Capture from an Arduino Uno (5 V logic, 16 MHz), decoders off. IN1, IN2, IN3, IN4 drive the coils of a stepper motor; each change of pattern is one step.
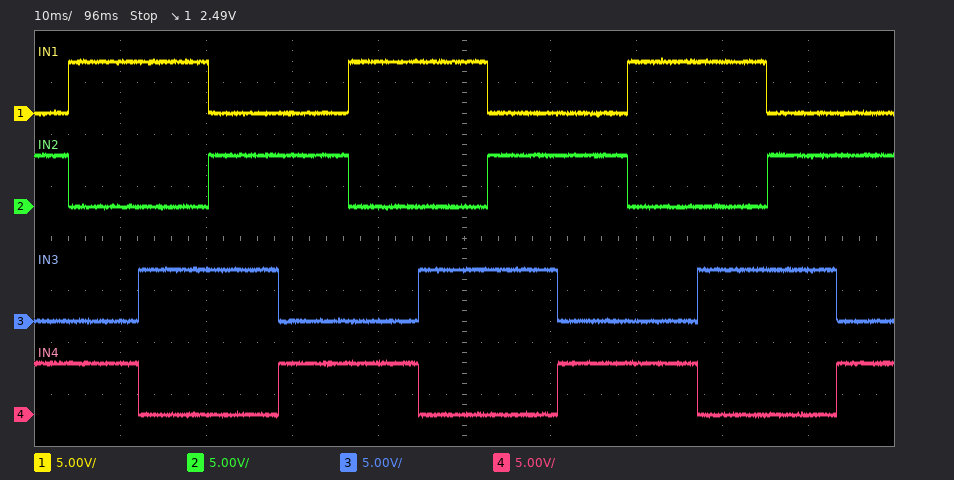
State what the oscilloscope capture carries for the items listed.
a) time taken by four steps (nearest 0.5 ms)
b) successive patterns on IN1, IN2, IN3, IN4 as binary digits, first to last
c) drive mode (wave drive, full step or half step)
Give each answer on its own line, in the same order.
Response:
32.5 ms
0101 1001 1010 0110 0101 1001 1010 0110 0101 1001 1010 0110 0101
full step
